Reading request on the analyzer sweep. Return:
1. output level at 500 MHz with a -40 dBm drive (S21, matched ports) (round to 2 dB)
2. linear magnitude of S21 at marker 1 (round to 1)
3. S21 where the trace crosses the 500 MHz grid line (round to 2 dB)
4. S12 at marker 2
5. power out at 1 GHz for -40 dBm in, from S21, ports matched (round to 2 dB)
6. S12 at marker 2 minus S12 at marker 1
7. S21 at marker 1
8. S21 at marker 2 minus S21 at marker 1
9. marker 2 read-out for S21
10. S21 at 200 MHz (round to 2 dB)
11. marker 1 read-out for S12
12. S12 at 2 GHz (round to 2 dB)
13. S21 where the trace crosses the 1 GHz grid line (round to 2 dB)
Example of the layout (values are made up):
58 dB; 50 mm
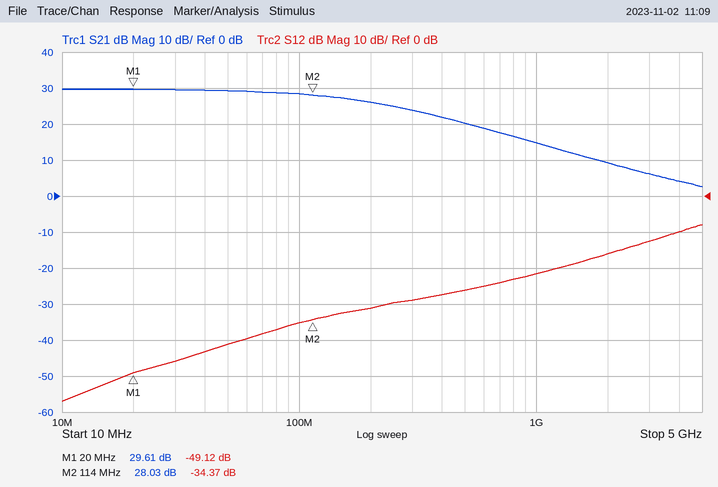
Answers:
-20 dBm; 30; 20 dB; -34.37 dB; -26 dBm; 14.75 dB; 29.61 dB; -1.58 dB; 28.03 dB; 26 dB; -49.12 dB; -16 dB; 14 dB
